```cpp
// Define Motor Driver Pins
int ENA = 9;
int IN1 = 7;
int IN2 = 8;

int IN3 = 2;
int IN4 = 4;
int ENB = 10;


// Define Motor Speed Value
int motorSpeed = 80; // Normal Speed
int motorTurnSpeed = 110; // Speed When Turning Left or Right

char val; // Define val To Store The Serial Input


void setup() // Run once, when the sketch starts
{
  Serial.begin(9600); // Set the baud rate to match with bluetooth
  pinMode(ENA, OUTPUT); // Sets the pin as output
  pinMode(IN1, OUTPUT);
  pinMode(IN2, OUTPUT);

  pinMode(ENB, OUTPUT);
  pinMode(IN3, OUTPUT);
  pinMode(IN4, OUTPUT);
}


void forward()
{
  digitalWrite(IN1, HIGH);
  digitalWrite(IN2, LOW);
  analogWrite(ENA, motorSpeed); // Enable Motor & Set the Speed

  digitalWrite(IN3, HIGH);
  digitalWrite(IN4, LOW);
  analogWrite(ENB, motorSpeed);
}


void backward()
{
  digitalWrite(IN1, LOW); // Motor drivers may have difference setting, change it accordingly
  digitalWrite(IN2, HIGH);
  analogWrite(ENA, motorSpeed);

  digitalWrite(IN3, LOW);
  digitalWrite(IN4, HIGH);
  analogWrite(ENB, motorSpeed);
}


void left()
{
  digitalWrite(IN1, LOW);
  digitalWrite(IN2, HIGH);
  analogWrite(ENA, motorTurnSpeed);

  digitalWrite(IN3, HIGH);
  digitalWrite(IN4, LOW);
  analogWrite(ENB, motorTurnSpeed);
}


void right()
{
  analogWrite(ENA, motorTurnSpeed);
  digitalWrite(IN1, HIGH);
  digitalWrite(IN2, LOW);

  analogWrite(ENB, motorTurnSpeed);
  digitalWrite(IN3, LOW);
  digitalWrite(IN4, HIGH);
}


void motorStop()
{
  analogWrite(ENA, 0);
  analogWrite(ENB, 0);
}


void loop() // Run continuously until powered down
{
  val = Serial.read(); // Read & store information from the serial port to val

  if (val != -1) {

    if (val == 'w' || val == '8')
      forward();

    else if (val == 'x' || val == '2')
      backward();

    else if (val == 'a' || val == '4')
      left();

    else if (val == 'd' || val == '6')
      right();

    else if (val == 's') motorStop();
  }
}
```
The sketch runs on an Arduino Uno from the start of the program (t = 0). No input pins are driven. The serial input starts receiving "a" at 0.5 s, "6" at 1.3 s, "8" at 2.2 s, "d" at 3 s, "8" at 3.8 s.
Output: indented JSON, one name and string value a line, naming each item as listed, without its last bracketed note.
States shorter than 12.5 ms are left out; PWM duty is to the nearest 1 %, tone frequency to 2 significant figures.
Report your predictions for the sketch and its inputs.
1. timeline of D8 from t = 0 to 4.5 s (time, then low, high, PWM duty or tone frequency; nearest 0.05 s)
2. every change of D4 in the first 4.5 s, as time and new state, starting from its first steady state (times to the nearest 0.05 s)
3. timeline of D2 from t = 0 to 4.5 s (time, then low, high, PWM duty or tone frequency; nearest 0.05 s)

{
  "timeline of D8 from t = 0 to 4.5 s": "0 s low; 0.5 s high; 1.3 s low",
  "every change of D4 in the first 4.5 s, as time and new state, starting from its first steady state": "0 s low; 1.3 s high; 2.2 s low; 3 s high; 3.8 s low",
  "timeline of D2 from t = 0 to 4.5 s": "0 s low; 0.5 s high; 1.3 s low; 2.2 s high; 3 s low; 3.8 s high"
}
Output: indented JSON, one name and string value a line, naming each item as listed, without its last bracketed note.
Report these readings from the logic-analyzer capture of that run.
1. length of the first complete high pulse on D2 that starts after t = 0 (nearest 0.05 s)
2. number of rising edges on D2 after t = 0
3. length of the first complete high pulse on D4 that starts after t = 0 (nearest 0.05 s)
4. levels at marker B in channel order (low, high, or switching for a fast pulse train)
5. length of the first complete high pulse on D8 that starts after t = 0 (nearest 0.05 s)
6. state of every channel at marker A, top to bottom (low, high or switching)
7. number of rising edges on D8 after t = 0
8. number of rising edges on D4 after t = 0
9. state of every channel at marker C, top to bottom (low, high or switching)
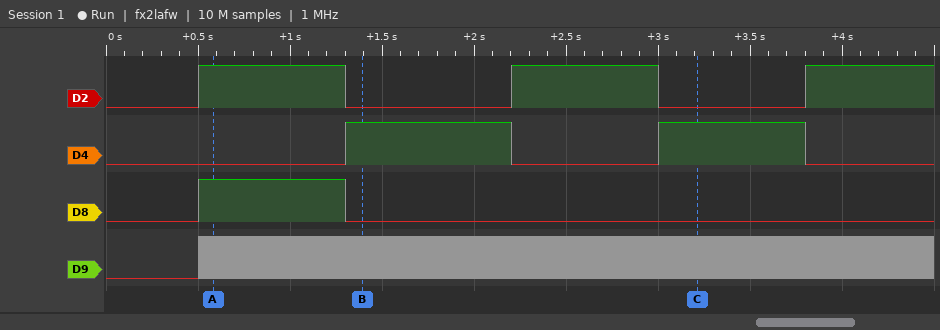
{
  "length of the first complete high pulse on D2 that starts after t = 0": "0.80 s",
  "number of rising edges on D2 after t = 0": "3",
  "length of the first complete high pulse on D4 that starts after t = 0": "0.90 s",
  "levels at marker B in channel order": "D2 low, D4 high, D8 low, D9 switching",
  "length of the first complete high pulse on D8 that starts after t = 0": "0.80 s",
  "state of every channel at marker A, top to bottom": "D2 high, D4 low, D8 high, D9 switching",
  "number of rising edges on D8 after t = 0": "1",
  "number of rising edges on D4 after t = 0": "2",
  "state of every channel at marker C, top to bottom": "D2 low, D4 high, D8 low, D9 switching"
}
